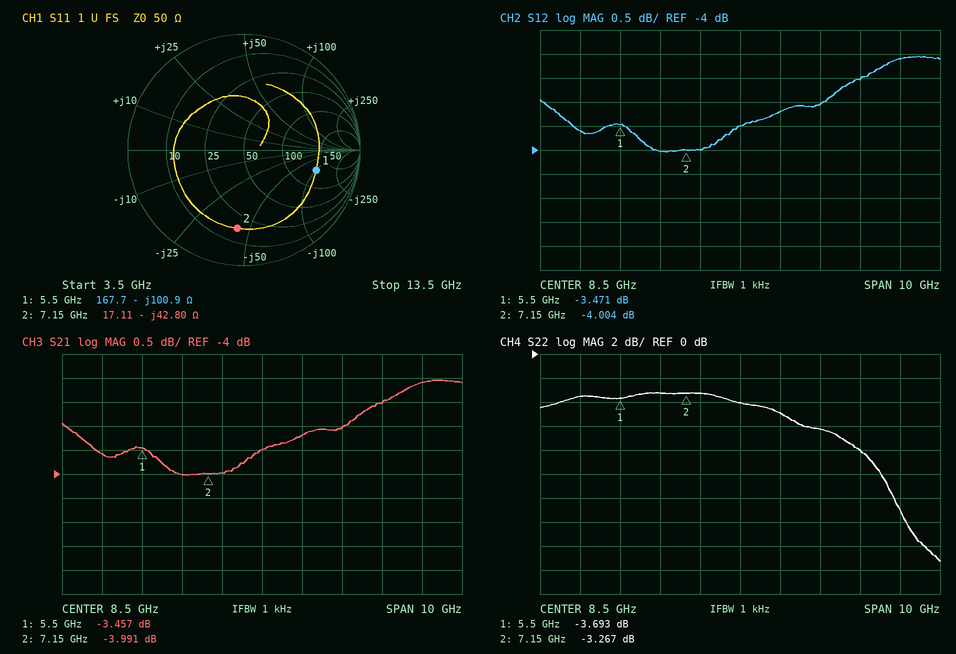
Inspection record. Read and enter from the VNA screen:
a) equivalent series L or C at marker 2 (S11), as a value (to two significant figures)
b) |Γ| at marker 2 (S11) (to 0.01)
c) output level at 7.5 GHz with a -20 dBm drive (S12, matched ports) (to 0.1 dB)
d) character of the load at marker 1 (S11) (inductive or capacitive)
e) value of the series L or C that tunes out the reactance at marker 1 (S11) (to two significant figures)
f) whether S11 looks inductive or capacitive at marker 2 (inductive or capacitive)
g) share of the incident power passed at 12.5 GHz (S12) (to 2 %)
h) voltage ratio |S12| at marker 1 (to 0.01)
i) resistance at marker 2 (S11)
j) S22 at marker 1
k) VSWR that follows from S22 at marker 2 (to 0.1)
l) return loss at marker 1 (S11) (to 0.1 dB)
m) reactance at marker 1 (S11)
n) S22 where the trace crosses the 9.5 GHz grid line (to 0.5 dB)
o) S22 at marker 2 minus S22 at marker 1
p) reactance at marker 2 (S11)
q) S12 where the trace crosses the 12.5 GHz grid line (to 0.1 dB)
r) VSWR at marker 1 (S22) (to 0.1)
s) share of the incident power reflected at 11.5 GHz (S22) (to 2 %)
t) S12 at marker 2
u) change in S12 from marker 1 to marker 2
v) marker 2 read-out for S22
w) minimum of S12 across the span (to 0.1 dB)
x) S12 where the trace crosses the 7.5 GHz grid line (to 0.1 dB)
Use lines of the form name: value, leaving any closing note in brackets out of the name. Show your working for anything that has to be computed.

equivalent series L or C at marker 2 (S11), as a value: C = 1/(2π × 7.15 GHz × 42.8 Ω) ≈ 520 fF
|Γ| at marker 2 (S11): 0.68
output level at 7.5 GHz with a -20 dBm drive (S12, matched ports): -20 dBm + (-4.0 dB) = -24.0 dBm
character of the load at marker 1 (S11): capacitive
value of the series L or C that tunes out the reactance at marker 1 (S11): L = 100.9 Ω/(2π × 5.5 GHz) ≈ 2.9 nH
whether S11 looks inductive or capacitive at marker 2: capacitive
share of the incident power passed at 12.5 GHz (S12): 10^(-2.1/10) ≈ 62 %
voltage ratio |S12| at marker 1: 10^(-3.471/20) ≈ 0.67
resistance at marker 2: 17.11 Ω
S22 at marker 1: -3.693 dB
VSWR that follows from S22 at marker 2: (1 + 0.6865)/(1 − 0.6865) ≈ 5.4
return loss at marker 1 (S11): 3.8 dB
reactance at marker 1: -100.9 Ω
S22 where the trace crosses the 9.5 GHz grid line: -5.0 dB
S22 at marker 2 minus S22 at marker 1: -3.267 − (-3.693) = 0.426 dB
reactance at marker 2: -42.80 Ω
S12 where the trace crosses the 12.5 GHz grid line: -2.1 dB
VSWR at marker 1 (S22): (1 + 0.6537)/(1 − 0.6537) ≈ 4.8
share of the incident power reflected at 11.5 GHz (S22): 10^(-8/10) ≈ 16 %
S12 at marker 2: -4.004 dB
change in S12 from marker 1 to marker 2: -4.004 − (-3.471) = -0.533 dB
marker 2 read-out for S22: -3.267 dB
minimum of S12 across the span: -4.0 dB
S12 where the trace crosses the 7.5 GHz grid line: -4.0 dB
